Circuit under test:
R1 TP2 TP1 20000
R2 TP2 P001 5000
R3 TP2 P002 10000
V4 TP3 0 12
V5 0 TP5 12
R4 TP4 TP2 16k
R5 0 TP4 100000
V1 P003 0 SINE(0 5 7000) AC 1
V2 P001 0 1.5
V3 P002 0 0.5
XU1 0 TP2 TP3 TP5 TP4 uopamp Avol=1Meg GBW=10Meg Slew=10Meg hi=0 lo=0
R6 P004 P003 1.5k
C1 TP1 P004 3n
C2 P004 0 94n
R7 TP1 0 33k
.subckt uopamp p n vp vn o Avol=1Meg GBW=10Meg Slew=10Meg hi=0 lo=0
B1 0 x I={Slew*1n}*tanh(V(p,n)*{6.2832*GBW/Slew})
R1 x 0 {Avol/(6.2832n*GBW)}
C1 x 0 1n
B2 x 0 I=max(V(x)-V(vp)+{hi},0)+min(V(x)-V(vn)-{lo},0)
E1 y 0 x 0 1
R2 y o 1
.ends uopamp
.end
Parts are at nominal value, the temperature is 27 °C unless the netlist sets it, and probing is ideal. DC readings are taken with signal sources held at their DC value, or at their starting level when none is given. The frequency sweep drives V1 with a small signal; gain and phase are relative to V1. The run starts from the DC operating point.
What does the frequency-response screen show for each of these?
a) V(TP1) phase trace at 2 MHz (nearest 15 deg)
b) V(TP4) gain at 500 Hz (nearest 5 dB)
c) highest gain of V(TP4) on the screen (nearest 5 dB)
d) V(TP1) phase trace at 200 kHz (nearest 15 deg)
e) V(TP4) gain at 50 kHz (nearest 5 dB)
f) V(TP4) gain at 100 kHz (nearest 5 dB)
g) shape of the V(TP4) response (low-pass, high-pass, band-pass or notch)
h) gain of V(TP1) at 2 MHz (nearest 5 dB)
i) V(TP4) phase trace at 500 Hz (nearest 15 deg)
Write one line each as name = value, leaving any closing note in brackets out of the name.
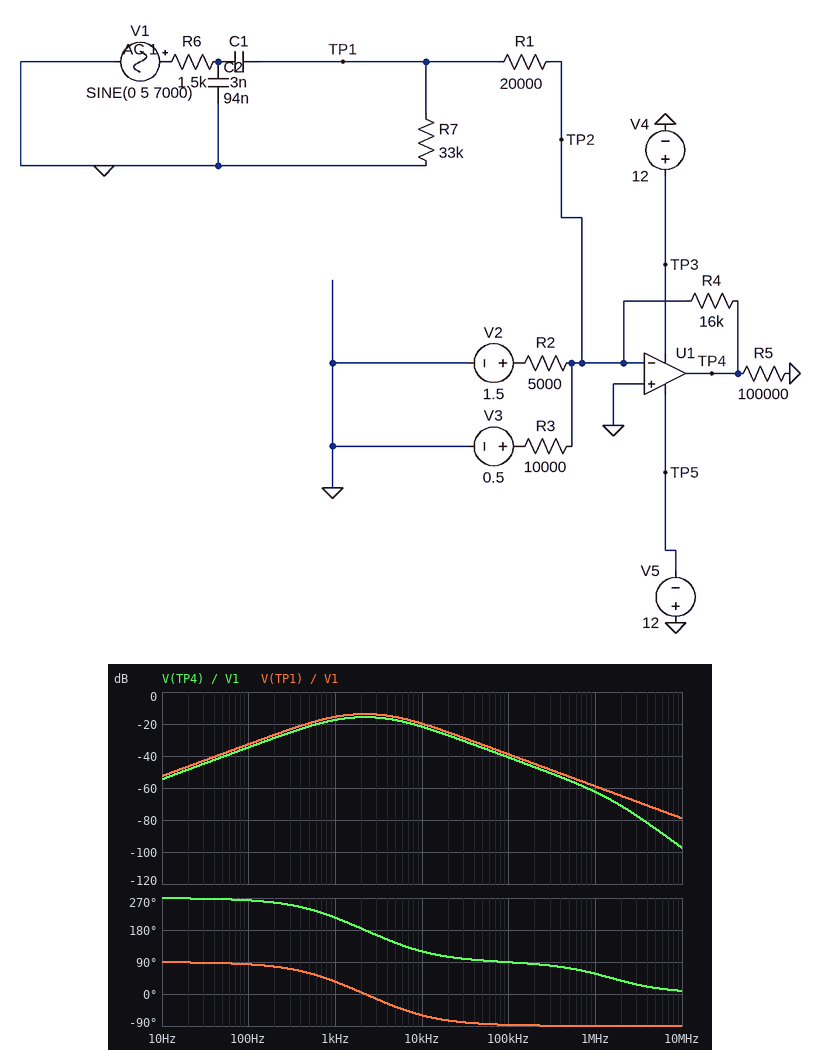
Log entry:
V(TP1) phase trace at 2 MHz = -90 deg
V(TP4) gain at 500 Hz = -20 dB
highest gain of V(TP4) on the screen = -15 dB
V(TP1) phase trace at 200 kHz = -90 deg
V(TP4) gain at 50 kHz = -35 dB
V(TP4) gain at 100 kHz = -40 dB
shape of the V(TP4) response = band-pass
gain of V(TP1) at 2 MHz = -65 dB
V(TP4) phase trace at 500 Hz = 240 deg
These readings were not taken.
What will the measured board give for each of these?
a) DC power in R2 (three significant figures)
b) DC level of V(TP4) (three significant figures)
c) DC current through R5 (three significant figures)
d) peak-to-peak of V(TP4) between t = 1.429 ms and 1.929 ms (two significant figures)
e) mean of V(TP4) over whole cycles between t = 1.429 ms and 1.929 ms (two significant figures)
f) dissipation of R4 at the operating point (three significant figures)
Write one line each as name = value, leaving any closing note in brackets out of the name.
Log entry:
DC power in R2 = 450 µW
DC level of V(TP4) = -5.60 V
DC current through R5 = 56.0 µA
peak-to-peak of V(TP4) between t = 1.429 ms and 1.929 ms = 1.1 V
mean of V(TP4) over whole cycles between t = 1.429 ms and 1.929 ms = -5.6 V
dissipation of R4 at the operating point = 1.96 mW
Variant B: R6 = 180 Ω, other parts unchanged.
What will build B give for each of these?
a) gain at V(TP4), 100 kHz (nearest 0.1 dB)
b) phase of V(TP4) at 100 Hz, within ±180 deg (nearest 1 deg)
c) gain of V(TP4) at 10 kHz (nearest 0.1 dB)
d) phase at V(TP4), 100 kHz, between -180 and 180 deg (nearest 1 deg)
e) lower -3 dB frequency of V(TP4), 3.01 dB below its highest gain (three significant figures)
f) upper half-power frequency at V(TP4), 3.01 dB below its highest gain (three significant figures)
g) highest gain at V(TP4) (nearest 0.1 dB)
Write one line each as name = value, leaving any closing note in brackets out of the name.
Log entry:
gain at V(TP4), 100 kHz = -22.5 dB
phase of V(TP4) at 100 Hz, within ±180 deg = -92 deg
gain of V(TP4) at 10 kHz = -6.0 dB
phase at V(TP4), 100 kHz, between -180 and 180 deg = 94 deg
lower -3 dB frequency of V(TP4), 3.01 dB below its highest gain = 2.46 kHz
upper half-power frequency at V(TP4), 3.01 dB below its highest gain = 16.3 kHz
highest gain at V(TP4) = -5.3 dB
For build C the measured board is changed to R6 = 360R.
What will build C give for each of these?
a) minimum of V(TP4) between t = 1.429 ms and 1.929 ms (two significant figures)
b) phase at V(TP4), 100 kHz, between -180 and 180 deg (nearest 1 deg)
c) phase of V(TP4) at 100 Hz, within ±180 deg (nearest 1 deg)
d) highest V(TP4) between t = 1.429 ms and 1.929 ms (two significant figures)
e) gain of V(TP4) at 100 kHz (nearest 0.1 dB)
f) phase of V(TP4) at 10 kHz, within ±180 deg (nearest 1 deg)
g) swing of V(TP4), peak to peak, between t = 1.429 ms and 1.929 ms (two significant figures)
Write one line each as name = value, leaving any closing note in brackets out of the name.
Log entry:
minimum of V(TP4) between t = 1.429 ms and 1.929 ms = -7.5 V
phase at V(TP4), 100 kHz, between -180 and 180 deg = 91 deg
phase of V(TP4) at 100 Hz, within ±180 deg = -93 deg
highest V(TP4) between t = 1.429 ms and 1.929 ms = -3.7 V
gain of V(TP4) at 100 kHz = -28.5 dB
phase of V(TP4) at 10 kHz, within ±180 deg = 138 deg
swing of V(TP4), peak to peak, between t = 1.429 ms and 1.929 ms = 3.8 V
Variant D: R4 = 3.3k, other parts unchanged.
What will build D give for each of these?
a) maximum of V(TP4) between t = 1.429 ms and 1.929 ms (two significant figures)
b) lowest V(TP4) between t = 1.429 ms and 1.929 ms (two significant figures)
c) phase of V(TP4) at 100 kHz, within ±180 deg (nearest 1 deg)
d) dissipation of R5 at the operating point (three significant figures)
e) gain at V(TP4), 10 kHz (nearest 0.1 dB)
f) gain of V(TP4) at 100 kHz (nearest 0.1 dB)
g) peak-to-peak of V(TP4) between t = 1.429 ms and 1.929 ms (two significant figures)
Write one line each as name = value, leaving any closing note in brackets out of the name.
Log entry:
maximum of V(TP4) between t = 1.429 ms and 1.929 ms = -1.0 V
lowest V(TP4) between t = 1.429 ms and 1.929 ms = -1.3 V
phase of V(TP4) at 100 kHz, within ±180 deg = 92 deg
dissipation of R5 at the operating point = 13.3 µW
gain at V(TP4), 10 kHz = -35.4 dB
gain of V(TP4) at 100 kHz = -54.6 dB
peak-to-peak of V(TP4) between t = 1.429 ms and 1.929 ms = 220 mV
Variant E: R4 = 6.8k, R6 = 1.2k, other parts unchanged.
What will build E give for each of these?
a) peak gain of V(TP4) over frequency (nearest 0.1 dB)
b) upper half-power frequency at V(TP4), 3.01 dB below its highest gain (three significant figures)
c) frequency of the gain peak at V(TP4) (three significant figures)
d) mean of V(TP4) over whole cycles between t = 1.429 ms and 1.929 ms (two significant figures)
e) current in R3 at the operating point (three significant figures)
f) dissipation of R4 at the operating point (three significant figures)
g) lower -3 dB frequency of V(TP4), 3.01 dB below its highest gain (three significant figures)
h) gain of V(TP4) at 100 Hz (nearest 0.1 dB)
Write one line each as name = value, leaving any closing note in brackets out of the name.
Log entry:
peak gain of V(TP4) over frequency = -21.7 dB
upper half-power frequency at V(TP4), 3.01 dB below its highest gain = 6.70 kHz
frequency of the gain peak at V(TP4) = 2.45 kHz
mean of V(TP4) over whole cycles between t = 1.429 ms and 1.929 ms = -2.4 V
current in R3 at the operating point = 50.0 µA
dissipation of R4 at the operating point = 833 µW
lower -3 dB frequency of V(TP4), 3.01 dB below its highest gain = 897 Hz
gain of V(TP4) at 100 Hz = -42.0 dB
